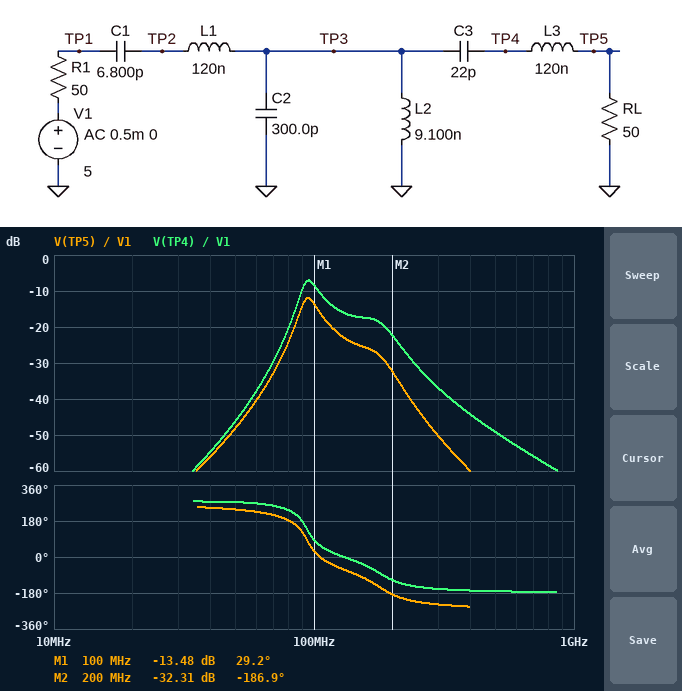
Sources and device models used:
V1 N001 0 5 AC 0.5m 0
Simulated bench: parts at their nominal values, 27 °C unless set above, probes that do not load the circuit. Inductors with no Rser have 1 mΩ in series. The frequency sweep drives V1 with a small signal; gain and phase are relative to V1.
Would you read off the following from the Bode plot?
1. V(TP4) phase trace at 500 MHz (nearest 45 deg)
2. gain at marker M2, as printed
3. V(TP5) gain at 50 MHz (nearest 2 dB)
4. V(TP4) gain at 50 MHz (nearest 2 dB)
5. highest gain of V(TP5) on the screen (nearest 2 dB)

-180 deg
-32.31 dB
-48 dB
-46 dB
-12 dB
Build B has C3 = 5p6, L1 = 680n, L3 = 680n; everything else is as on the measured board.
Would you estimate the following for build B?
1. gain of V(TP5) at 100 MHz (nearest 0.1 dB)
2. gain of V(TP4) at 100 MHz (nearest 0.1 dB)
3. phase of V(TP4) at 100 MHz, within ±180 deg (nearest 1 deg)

-8.3 dB
10.4 dB
-99 deg
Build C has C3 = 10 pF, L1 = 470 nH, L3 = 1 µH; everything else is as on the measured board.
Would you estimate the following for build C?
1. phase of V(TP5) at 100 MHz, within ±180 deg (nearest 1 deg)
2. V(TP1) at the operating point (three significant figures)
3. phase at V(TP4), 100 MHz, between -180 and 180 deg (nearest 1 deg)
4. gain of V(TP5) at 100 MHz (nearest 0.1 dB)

-146 deg
5.00 V
-61 deg
-16.0 dB
